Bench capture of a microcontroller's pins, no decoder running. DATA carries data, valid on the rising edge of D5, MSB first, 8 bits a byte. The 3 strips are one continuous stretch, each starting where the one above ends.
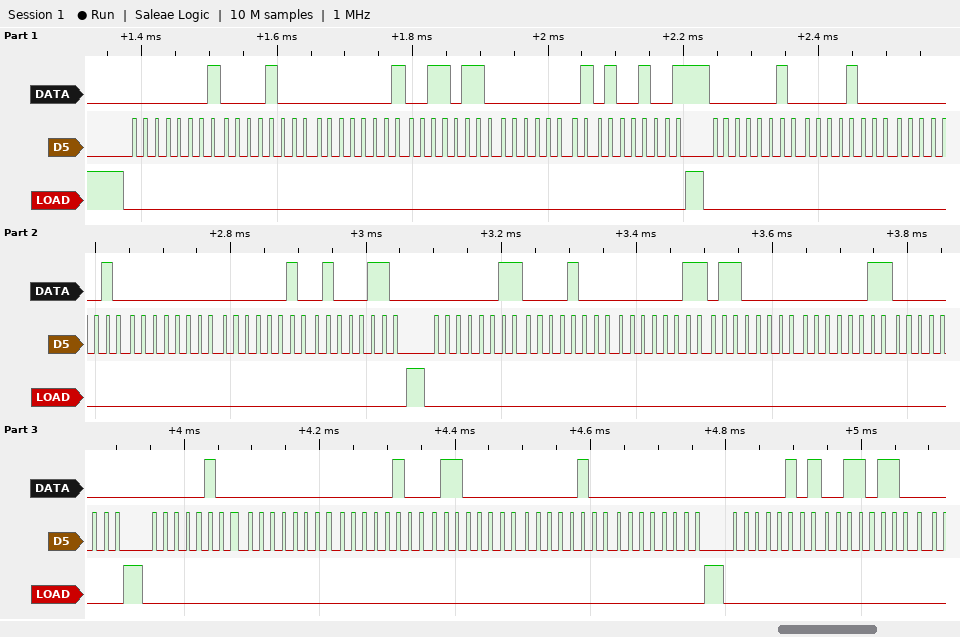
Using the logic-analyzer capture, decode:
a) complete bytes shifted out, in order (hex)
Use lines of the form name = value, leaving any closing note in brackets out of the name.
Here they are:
complete bytes shifted out, in order = 01 08 01 36 01 49 02 08 02 00 02 46 03 08 03 60 03 00 04 00 04 60 04 00 05 36
